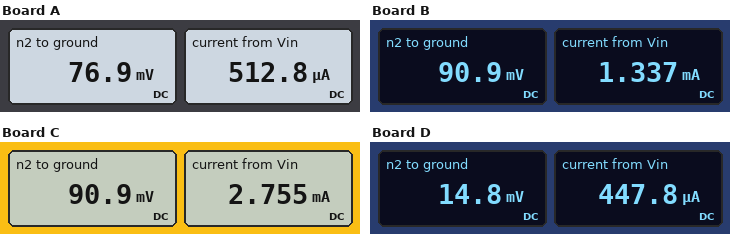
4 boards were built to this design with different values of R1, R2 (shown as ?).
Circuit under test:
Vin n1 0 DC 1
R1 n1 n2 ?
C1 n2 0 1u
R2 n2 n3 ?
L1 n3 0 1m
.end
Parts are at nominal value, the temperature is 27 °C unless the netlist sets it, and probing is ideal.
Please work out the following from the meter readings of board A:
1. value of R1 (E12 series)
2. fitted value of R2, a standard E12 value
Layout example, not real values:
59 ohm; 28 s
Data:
1.8 kΩ; 150 Ω
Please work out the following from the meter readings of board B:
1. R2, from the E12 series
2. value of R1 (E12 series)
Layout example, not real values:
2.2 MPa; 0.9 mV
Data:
68 Ω; 680 Ω
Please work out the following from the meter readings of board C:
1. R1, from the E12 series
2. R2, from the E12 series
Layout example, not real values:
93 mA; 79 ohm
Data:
330 Ω; 33 Ω
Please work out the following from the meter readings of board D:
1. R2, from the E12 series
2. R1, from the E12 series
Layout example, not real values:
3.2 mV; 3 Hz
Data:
33 Ω; 2.2 kΩ
